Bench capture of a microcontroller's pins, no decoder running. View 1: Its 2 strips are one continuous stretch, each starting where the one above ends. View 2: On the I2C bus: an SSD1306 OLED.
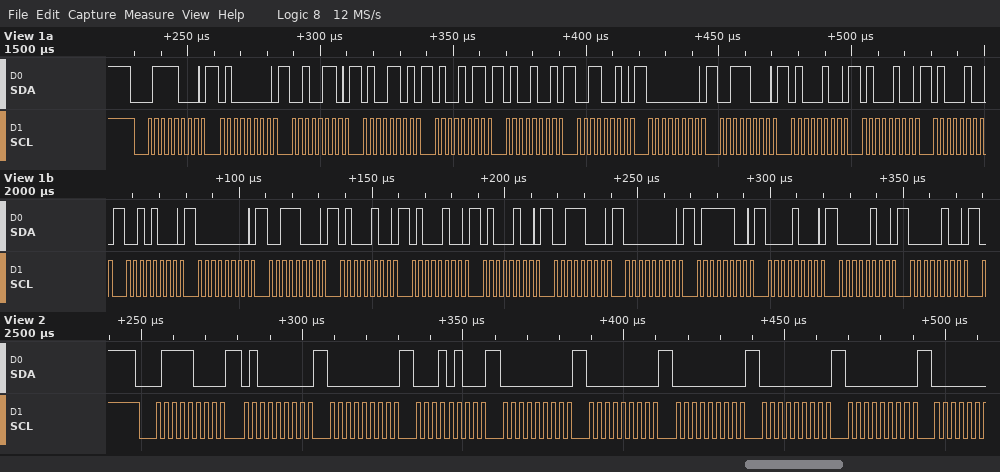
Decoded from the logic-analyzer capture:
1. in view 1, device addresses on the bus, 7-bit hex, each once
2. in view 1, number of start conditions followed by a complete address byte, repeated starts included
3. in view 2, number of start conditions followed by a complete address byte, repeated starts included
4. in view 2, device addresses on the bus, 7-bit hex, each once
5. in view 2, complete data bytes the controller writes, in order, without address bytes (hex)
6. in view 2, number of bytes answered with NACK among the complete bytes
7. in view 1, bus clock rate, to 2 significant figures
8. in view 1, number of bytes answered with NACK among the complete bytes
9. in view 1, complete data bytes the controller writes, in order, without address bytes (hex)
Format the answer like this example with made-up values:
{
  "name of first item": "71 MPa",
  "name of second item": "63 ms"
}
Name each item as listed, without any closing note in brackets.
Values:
{
  "in view 1, device addresses on the bus, 7-bit hex, each once": "0x3C",
  "in view 1, number of start conditions followed by a complete address byte, repeated starts included": "1",
  "in view 2, number of start conditions followed by a complete address byte, repeated starts included": "1",
  "in view 2, device addresses on the bus, 7-bit hex, each once": "0x3C",
  "in view 2, complete data bytes the controller writes, in order, without address bytes": "40 00 14 00 00 00 00 00",
  "in view 2, number of bytes answered with NACK among the complete bytes": "0",
  "in view 1, bus clock rate, to 2 significant figures": "400 kHz",
  "in view 1, number of bytes answered with NACK among the complete bytes": "0",
  "in view 1, complete data bytes the controller writes, in order, without address bytes": "40 26 4D 4B 49 32 00 38 44 44 44 28 00 38 44 44 44 38 00 7C 08 04 04"
}
